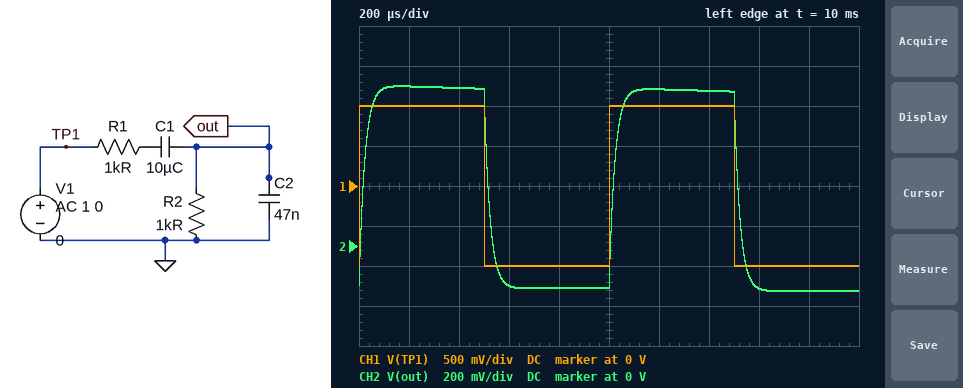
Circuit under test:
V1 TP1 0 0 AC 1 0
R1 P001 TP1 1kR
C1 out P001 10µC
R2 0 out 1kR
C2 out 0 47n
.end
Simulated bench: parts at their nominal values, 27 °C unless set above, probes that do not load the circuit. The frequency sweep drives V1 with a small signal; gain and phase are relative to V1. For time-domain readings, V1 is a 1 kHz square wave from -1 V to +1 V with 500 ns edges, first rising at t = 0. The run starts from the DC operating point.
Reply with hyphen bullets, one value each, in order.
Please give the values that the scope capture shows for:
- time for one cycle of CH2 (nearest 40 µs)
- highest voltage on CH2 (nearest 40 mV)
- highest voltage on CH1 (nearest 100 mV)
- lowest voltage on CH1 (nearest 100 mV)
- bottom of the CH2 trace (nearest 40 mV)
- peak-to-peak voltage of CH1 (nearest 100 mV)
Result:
- 1.00 ms
- 800 mV
- 1.0 V
- -1.0 V
- -240 mV
- 2.0 V
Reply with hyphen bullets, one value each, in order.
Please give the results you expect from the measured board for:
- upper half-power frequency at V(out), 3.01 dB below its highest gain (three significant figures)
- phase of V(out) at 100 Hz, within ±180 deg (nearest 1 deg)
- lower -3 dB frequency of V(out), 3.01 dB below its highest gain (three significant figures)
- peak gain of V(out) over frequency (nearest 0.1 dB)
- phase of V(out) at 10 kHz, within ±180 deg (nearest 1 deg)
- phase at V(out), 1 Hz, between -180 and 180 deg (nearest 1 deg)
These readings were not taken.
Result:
- 6.80 kHz
- 4 deg
- 7.93 Hz
- -6.0 dB
- -56 deg
- 83 deg
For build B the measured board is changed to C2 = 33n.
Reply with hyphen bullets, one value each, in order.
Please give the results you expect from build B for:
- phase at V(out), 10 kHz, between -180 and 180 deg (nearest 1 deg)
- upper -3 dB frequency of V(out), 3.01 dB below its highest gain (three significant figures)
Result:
- -46 deg
- 9.67 kHz
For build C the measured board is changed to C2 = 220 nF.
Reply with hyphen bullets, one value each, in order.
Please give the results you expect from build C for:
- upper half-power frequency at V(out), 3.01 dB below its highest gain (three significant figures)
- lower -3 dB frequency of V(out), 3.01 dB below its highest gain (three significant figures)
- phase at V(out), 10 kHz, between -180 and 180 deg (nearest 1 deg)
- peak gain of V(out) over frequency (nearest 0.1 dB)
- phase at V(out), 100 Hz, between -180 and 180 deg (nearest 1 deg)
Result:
- 1.47 kHz
- 7.83 Hz
- -82 deg
- -6.1 dB
- 1 deg
